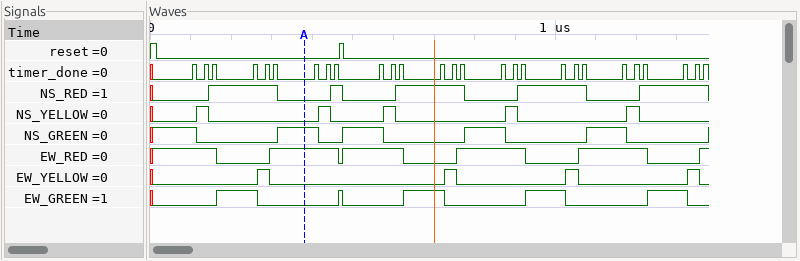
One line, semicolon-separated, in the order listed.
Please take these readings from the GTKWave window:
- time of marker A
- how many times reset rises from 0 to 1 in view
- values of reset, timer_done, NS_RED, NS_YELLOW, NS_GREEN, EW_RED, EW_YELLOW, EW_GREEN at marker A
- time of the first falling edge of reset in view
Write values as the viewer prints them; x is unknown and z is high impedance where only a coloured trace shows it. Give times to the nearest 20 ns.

380 ns; 1; reset=0, timer_done=0, NS_RED=0, NS_YELLOW=0, NS_GREEN=1, EW_RED=1, EW_YELLOW=0, EW_GREEN=0; 20 ns
